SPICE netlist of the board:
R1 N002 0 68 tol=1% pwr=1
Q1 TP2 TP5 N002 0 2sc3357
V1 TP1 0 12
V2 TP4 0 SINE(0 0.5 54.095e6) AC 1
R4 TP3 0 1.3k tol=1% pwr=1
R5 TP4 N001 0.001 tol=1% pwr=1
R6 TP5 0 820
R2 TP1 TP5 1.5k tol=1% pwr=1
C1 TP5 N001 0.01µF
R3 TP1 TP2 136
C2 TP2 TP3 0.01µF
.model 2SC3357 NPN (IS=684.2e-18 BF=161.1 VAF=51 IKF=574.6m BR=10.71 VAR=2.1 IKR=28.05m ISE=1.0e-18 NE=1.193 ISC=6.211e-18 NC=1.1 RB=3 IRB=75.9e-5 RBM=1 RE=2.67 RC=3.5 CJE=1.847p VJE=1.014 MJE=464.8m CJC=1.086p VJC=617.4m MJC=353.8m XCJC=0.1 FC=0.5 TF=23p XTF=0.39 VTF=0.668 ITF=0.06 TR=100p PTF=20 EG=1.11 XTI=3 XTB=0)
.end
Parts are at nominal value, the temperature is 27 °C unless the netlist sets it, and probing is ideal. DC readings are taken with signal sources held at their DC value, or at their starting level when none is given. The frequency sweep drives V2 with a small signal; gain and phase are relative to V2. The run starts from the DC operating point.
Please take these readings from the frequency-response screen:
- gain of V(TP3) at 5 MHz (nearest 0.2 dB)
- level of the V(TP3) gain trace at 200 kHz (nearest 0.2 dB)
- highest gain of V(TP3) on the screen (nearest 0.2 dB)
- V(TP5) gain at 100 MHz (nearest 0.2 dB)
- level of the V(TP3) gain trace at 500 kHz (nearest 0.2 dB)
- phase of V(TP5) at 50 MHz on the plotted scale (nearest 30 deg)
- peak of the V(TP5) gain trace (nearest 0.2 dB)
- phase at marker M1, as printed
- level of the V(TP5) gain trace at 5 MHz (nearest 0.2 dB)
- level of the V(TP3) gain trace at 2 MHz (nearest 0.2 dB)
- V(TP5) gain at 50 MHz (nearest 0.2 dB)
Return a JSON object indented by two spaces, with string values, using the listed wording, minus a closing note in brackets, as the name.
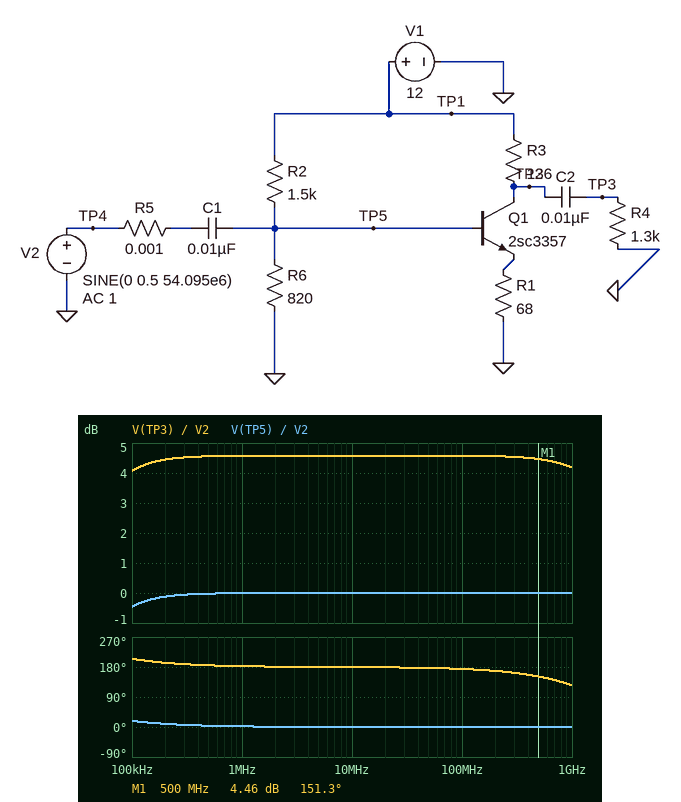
{
  "gain of V(TP3) at 5 MHz": "4.6 dB",
  "level of the V(TP3) gain trace at 200 kHz": "4.4 dB",
  "highest gain of V(TP3) on the screen": "4.6 dB",
  "V(TP5) gain at 100 MHz": "0 dB",
  "level of the V(TP3) gain trace at 500 kHz": "4.6 dB",
  "phase of V(TP5) at 50 MHz on the plotted scale": "0 deg",
  "peak of the V(TP5) gain trace": "0 dB",
  "phase at marker M1, as printed": "151.3 deg",
  "level of the V(TP5) gain trace at 5 MHz": "0 dB",
  "level of the V(TP3) gain trace at 2 MHz": "4.6 dB",
  "V(TP5) gain at 50 MHz": "0 dB"
}
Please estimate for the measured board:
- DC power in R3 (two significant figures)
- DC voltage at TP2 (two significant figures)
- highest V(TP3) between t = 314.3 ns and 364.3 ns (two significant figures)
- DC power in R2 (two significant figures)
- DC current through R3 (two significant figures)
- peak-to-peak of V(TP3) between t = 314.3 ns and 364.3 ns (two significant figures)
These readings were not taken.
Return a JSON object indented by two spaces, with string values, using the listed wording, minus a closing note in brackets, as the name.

{
  "DC power in R3": "260 mW",
  "DC voltage at TP2": "6.0 V",
  "highest V(TP3) between t = 314.3 ns and 364.3 ns": "850 mV",
  "DC power in R2": "43 mW",
  "DC current through R3": "44 mA",
  "peak-to-peak of V(TP3) between t = 314.3 ns and 364.3 ns": "1.7 V"
}
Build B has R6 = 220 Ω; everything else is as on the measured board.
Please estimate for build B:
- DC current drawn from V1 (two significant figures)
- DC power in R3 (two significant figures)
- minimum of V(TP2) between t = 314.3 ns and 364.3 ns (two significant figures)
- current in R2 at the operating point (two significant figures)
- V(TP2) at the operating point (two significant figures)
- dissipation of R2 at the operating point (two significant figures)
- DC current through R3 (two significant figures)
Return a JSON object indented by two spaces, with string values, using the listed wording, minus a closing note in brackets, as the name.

{
  "DC current drawn from V1": "17 mA",
  "DC power in R3": "14 mW",
  "minimum of V(TP2) between t = 314.3 ns and 364.3 ns": "9.8 V",
  "current in R2 at the operating point": "7.0 mA",
  "V(TP2) at the operating point": "11 V",
  "dissipation of R2 at the operating point": "73 mW",
  "DC current through R3": "10 mA"
}
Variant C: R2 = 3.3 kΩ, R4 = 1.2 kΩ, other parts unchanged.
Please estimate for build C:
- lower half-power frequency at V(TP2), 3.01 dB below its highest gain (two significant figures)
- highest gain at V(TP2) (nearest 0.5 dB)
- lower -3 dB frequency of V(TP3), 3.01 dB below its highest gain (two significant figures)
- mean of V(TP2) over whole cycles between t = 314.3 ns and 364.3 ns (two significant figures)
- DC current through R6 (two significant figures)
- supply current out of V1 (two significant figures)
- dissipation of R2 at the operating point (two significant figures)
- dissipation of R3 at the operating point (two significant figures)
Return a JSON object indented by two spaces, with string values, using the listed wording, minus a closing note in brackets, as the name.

{
  "lower half-power frequency at V(TP2), 3.01 dB below its highest gain": "25 kHz",
  "highest gain at V(TP2)": "4.5 dB",
  "lower -3 dB frequency of V(TP3), 3.01 dB below its highest gain": "31 kHz",
  "mean of V(TP2) over whole cycles between t = 314.3 ns and 364.3 ns": "9.2 V",
  "DC current through R6": "2.8 mA",
  "supply current out of V1": "23 mA",
  "dissipation of R2 at the operating point": "29 mW",
  "dissipation of R3 at the operating point": "57 mW"
}
